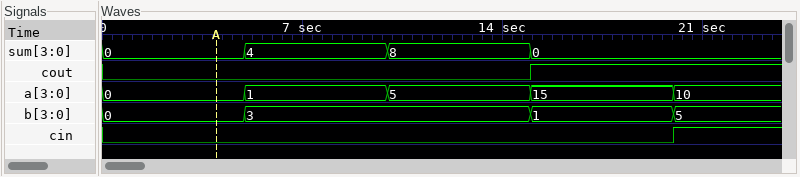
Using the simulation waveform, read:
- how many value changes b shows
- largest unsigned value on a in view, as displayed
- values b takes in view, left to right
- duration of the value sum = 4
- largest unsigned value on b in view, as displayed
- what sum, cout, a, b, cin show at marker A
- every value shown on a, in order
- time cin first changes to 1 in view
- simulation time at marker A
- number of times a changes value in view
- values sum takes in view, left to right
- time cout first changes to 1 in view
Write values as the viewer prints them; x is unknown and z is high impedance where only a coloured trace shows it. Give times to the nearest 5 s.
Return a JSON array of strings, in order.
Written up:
["3", "15", "0, 3, 1, 5", "5 s", "5", "sum=0, cout=0, a=0, b=0, cin=0", "0, 1, 5, 15, 10", "20 s", "5 s", "4", "0, 4, 8, 0", "15 s"]
